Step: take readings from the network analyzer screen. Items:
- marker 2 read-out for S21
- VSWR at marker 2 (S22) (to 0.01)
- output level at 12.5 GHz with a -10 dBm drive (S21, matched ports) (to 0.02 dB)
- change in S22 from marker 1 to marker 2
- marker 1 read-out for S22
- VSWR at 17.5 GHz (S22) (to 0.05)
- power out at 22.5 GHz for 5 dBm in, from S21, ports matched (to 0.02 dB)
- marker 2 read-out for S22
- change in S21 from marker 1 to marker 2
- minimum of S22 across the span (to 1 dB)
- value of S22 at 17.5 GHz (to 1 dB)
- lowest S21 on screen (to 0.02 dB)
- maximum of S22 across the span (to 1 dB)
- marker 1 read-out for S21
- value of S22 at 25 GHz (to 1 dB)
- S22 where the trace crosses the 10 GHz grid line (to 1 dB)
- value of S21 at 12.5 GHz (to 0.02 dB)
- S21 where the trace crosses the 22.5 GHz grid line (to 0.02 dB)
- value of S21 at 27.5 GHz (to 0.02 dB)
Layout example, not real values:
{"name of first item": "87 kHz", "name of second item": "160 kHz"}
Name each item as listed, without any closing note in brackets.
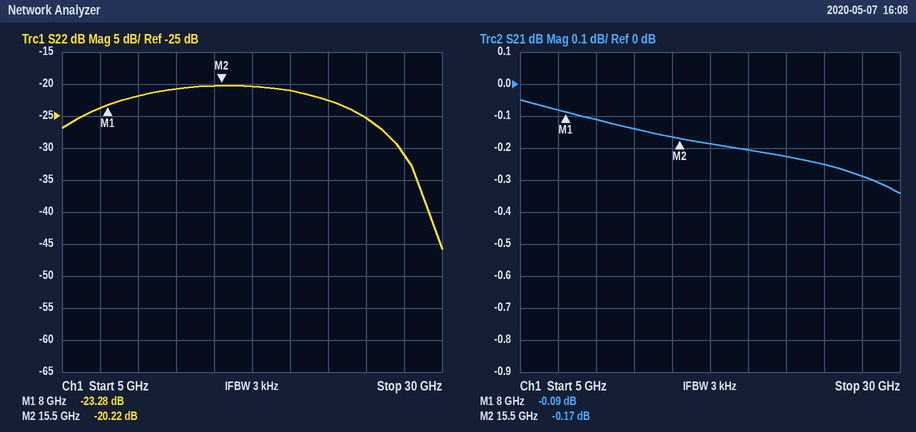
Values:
{"marker 2 read-out for S21": "-0.17 dB", "VSWR at marker 2 (S22)": "1.22", "output level at 12.5 GHz with a -10 dBm drive (S21, matched ports)": "-10.14 dBm", "change in S22 from marker 1 to marker 2": "3.06 dB", "marker 1 read-out for S22": "-23.28 dB", "VSWR at 17.5 GHz (S22)": "1.20", "power out at 22.5 GHz for 5 dBm in, from S21, ports matched": "4.78 dBm", "marker 2 read-out for S22": "-20.22 dB", "change in S21 from marker 1 to marker 2": "-0.08 dB", "minimum of S22 across the span": "-46 dB", "value of S22 at 17.5 GHz": "-20 dB", "lowest S21 on screen": "-0.34 dB", "maximum of S22 across the span": "-20 dB", "marker 1 read-out for S21": "-0.09 dB", "value of S22 at 25 GHz": "-25 dB", "S22 where the trace crosses the 10 GHz grid line": "-22 dB", "value of S21 at 12.5 GHz": "-0.14 dB", "S21 where the trace crosses the 22.5 GHz grid line": "-0.22 dB", "value of S21 at 27.5 GHz": "-0.28 dB"}
